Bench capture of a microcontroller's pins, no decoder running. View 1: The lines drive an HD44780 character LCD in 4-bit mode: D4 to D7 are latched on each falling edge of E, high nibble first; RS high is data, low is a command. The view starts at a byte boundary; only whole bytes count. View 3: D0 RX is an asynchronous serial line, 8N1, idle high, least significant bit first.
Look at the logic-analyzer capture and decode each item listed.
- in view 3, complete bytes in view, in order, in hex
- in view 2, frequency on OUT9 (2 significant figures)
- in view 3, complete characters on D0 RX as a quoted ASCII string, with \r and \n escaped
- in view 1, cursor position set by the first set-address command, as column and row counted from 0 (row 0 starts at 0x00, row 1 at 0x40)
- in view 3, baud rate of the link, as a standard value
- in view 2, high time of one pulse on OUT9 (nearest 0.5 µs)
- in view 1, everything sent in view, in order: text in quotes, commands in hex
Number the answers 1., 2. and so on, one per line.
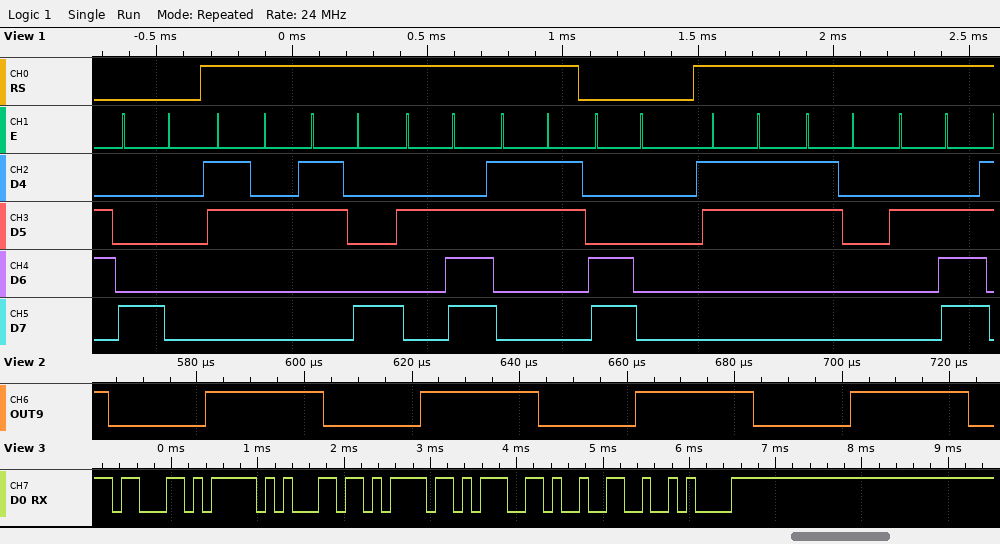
1. 63 5F 6C 6F 67 32 0A
2. 25 kHz
3. "c_log2\n"
4. column 0, row 0
5. 9600 baud
6. 22.0 µs
7. 0x80 "28.3" 0xC0 "30."
